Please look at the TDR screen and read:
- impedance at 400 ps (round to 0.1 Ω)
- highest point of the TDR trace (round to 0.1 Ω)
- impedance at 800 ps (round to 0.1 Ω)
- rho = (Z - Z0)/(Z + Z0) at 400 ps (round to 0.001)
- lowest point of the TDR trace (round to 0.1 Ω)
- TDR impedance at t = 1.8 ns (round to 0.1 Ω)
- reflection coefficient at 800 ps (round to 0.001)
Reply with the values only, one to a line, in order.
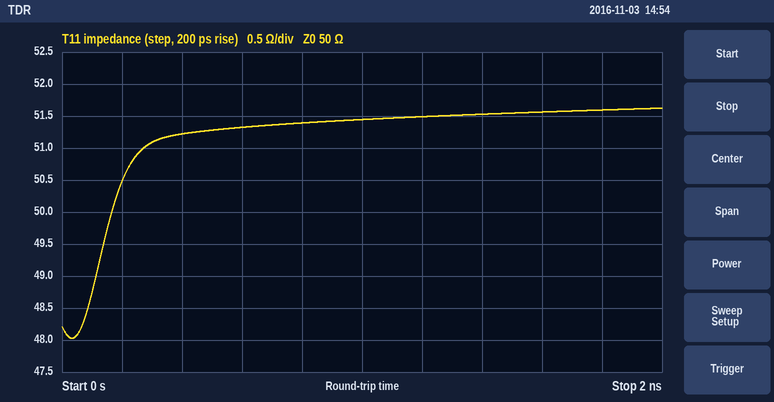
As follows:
51.2 Ω
51.6 Ω
51.4 Ω
+0.012
48.0 Ω
51.6 Ω
+0.014
